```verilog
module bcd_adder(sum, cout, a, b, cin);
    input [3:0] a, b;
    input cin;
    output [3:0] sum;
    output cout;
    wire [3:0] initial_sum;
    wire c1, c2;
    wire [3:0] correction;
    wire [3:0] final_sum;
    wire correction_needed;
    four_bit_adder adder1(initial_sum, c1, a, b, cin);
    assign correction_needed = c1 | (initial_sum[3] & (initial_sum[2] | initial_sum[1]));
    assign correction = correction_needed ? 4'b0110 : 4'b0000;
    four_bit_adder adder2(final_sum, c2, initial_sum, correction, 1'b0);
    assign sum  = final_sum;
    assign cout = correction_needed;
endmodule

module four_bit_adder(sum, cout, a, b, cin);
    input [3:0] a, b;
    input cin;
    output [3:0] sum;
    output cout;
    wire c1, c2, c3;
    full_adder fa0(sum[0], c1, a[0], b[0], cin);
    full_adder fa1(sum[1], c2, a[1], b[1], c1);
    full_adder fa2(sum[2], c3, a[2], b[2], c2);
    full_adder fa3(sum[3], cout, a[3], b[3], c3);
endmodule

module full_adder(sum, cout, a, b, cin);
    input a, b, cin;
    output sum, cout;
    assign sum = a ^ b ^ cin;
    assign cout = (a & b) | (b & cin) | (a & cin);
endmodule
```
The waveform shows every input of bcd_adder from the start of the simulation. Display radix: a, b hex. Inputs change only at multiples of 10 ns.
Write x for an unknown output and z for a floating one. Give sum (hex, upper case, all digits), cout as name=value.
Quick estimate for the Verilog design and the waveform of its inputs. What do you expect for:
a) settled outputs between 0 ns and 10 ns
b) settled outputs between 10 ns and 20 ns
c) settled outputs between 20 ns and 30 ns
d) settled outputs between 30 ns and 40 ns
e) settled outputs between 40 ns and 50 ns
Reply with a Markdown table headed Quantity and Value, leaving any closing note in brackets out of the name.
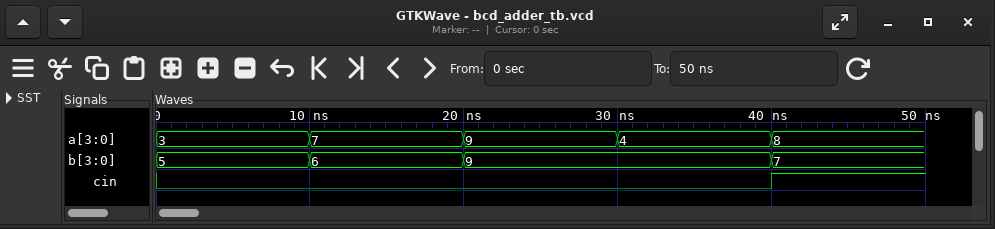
| Quantity | Value |
|---|---|
| settled outputs between 0 ns and 10 ns | sum=8, cout=0 |
| settled outputs between 10 ns and 20 ns | sum=3, cout=1 |
| settled outputs between 20 ns and 30 ns | sum=8, cout=1 |
| settled outputs between 30 ns and 40 ns | sum=3, cout=1 |
| settled outputs between 40 ns and 50 ns | sum=6, cout=1 |
